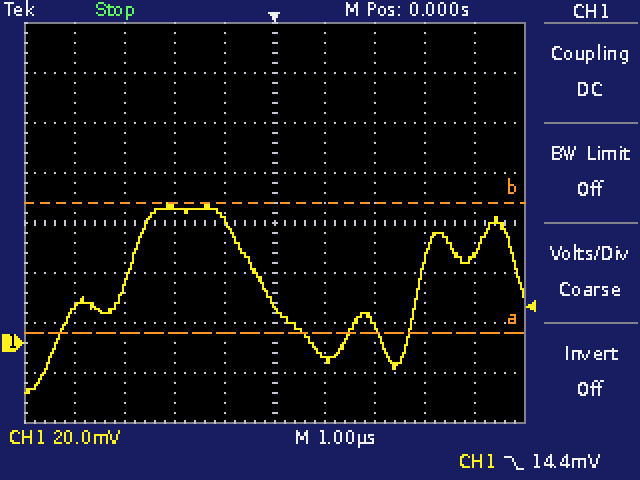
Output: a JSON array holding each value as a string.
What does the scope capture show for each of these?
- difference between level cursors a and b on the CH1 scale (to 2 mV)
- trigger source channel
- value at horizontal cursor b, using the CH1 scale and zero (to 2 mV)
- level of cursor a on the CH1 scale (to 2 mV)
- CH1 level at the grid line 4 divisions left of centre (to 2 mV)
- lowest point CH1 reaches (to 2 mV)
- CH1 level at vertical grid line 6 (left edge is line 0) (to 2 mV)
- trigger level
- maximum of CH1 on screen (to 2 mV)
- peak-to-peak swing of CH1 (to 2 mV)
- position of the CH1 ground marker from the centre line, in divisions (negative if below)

["52 mV", "CH1", "56 mV", "4 mV", "14 mV", "-20 mV", "-6 mV", "14.4 mV", "56 mV", "76 mV", "-2.4 div"]
